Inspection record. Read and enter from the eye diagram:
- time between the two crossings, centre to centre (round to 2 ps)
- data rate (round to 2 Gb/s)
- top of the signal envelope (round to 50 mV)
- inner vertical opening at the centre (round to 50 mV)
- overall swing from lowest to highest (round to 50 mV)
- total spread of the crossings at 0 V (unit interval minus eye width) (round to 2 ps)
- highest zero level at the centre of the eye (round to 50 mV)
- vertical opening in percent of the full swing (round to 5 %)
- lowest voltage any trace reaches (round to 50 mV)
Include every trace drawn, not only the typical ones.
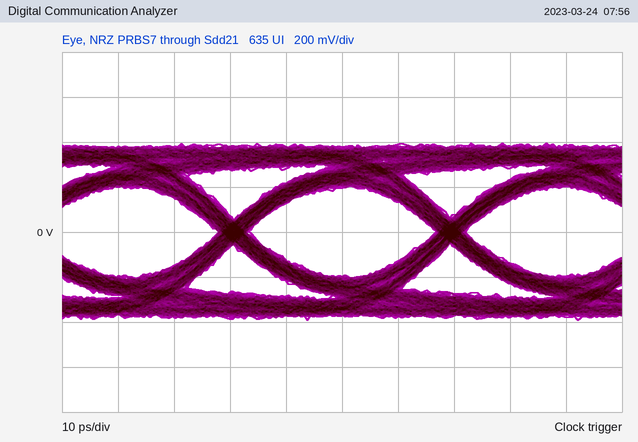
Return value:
38 ps
26 Gb/s
400 mV
400 mV
800 mV
6 ps
-200 mV
50 %
-400 mV
